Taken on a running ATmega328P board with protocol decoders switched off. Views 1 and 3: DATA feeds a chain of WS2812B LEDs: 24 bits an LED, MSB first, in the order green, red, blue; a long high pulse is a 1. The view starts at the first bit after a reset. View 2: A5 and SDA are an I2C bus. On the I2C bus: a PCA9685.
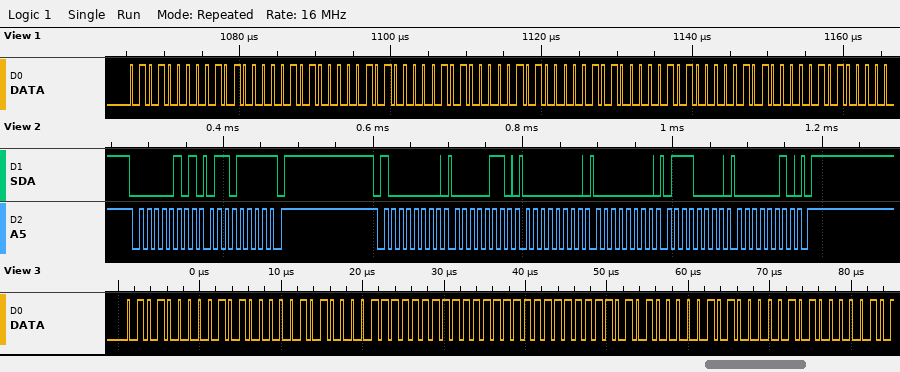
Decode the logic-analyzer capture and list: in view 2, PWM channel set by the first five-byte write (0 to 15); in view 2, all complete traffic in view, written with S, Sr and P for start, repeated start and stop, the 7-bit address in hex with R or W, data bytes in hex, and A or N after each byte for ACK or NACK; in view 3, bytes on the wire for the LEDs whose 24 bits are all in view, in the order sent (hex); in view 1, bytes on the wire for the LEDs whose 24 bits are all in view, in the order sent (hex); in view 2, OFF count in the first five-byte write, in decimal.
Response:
0
S 02R A 6F N P S 40W A 06 A 00 A 00 A 70 A 02 A P
50 50 50 FF FF FF 50 50 50
50 50 50 50 50 50 50 50 50
624
